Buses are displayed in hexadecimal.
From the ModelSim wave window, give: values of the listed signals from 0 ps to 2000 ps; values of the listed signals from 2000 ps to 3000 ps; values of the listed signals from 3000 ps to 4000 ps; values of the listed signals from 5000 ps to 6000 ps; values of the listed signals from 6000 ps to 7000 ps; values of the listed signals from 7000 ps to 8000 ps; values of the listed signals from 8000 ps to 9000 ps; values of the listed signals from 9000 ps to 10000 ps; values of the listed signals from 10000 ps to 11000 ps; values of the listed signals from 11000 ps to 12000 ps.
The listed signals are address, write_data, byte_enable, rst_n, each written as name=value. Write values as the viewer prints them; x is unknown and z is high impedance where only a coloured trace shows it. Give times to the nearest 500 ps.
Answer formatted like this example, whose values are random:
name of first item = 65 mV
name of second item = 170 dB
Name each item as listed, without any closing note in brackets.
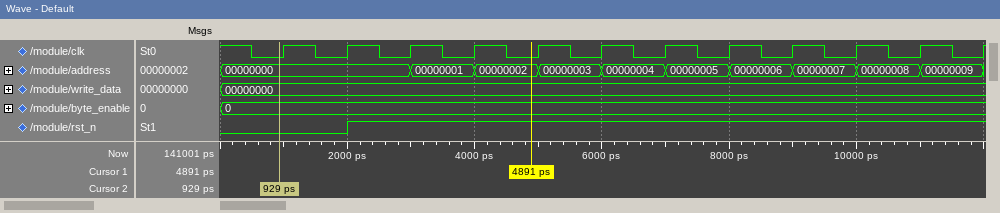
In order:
values of the listed signals from 0 ps to 2000 ps = address=00000000, write_data=00000000, byte_enable=0, rst_n=0
values of the listed signals from 2000 ps to 3000 ps = address=00000000, write_data=00000000, byte_enable=0, rst_n=1
values of the listed signals from 3000 ps to 4000 ps = address=00000001, write_data=00000000, byte_enable=0, rst_n=1
values of the listed signals from 5000 ps to 6000 ps = address=00000003, write_data=00000000, byte_enable=0, rst_n=1
values of the listed signals from 6000 ps to 7000 ps = address=00000004, write_data=00000000, byte_enable=0, rst_n=1
values of the listed signals from 7000 ps to 8000 ps = address=00000005, write_data=00000000, byte_enable=0, rst_n=1
values of the listed signals from 8000 ps to 9000 ps = address=00000006, write_data=00000000, byte_enable=0, rst_n=1
values of the listed signals from 9000 ps to 10000 ps = address=00000007, write_data=00000000, byte_enable=0, rst_n=1
values of the listed signals from 10000 ps to 11000 ps = address=00000008, write_data=00000000, byte_enable=0, rst_n=1
values of the listed signals from 11000 ps to 12000 ps = address=00000009, write_data=00000000, byte_enable=0, rst_n=1
